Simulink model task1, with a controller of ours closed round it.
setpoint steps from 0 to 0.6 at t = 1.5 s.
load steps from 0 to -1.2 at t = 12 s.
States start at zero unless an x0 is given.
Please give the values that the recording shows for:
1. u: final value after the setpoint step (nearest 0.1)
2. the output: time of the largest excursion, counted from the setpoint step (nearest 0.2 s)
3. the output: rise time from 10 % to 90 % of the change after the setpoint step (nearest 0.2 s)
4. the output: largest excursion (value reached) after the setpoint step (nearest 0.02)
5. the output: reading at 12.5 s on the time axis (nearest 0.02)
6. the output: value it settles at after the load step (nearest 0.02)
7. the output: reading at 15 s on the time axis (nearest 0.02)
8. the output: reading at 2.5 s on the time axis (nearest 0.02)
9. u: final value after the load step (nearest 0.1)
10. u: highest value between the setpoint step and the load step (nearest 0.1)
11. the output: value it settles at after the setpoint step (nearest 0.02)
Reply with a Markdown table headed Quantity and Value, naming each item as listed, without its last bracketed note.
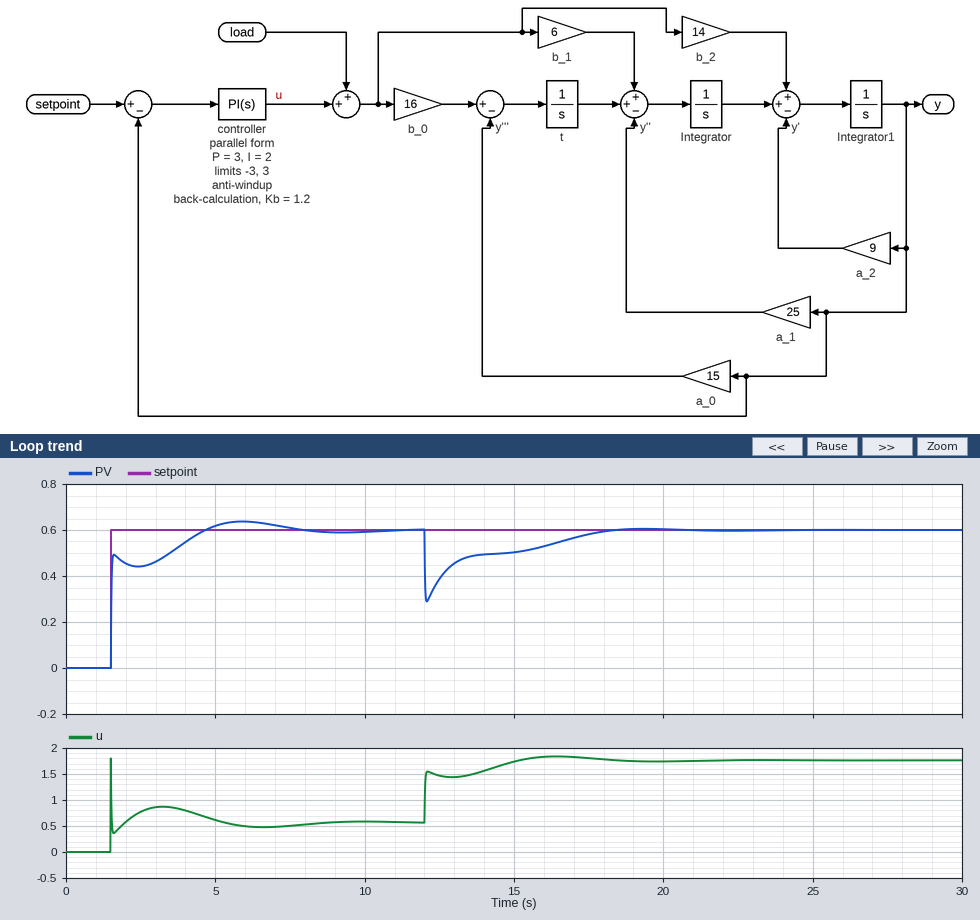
| Quantity | Value |
|---|---|
| u: final value after the setpoint step | 0.6 |
| the output: time of the largest excursion, counted from the setpoint step | 4.4 s |
| the output: rise time from 10 % to 90 % of the change after the setpoint step | 2.4 s |
| the output: largest excursion (value reached) after the setpoint step | 0.64 |
| the output: reading at 12.5 s on the time axis | 0.38 |
| the output: value it settles at after the load step | 0.60 |
| the output: reading at 15 s on the time axis | 0.50 |
| the output: reading at 2.5 s on the time axis | 0.44 |
| u: final value after the load step | 1.8 |
| u: highest value between the setpoint step and the load step | 1.8 |
| the output: value it settles at after the setpoint step | 0.60 |
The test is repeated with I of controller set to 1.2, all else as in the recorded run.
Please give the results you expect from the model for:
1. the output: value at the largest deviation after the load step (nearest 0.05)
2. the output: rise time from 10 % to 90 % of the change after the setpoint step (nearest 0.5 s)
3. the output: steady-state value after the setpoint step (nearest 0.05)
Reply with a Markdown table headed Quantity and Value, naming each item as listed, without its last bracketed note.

| Quantity | Value |
|---|---|
| the output: value at the largest deviation after the load step | 0.30 |
| the output: rise time from 10 % to 90 % of the change after the setpoint step | 3.0 s |
| the output: steady-state value after the setpoint step | 0.60 |
